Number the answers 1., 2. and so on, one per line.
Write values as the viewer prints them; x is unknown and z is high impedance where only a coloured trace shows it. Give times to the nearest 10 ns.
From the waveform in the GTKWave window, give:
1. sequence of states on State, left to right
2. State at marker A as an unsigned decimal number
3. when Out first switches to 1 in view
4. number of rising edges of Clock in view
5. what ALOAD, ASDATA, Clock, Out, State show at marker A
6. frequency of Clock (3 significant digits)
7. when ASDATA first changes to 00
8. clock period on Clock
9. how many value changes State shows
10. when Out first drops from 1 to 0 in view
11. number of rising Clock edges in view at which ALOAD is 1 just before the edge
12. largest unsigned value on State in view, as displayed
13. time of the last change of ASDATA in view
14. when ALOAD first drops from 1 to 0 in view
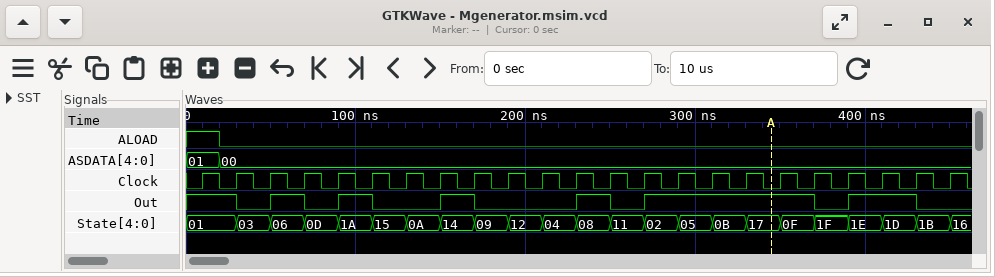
1. 01, 03, 06, 0D, 1A, 15, 0A, 14, 09, 12, 04, 08, 11, 02, 05, 0B, 17, 0F, 1F, 1E, 1D, 1B, 16
2. 23
3. 50 ns
4. 23
5. ALOAD=0, ASDATA=00, Clock=0, Out=1, State=17
6. 50.0 MHz
7. 20 ns
8. 20 ns
9. 22
10. 30 ns
11. 1
12. 1F
13. 20 ns
14. 20 ns
